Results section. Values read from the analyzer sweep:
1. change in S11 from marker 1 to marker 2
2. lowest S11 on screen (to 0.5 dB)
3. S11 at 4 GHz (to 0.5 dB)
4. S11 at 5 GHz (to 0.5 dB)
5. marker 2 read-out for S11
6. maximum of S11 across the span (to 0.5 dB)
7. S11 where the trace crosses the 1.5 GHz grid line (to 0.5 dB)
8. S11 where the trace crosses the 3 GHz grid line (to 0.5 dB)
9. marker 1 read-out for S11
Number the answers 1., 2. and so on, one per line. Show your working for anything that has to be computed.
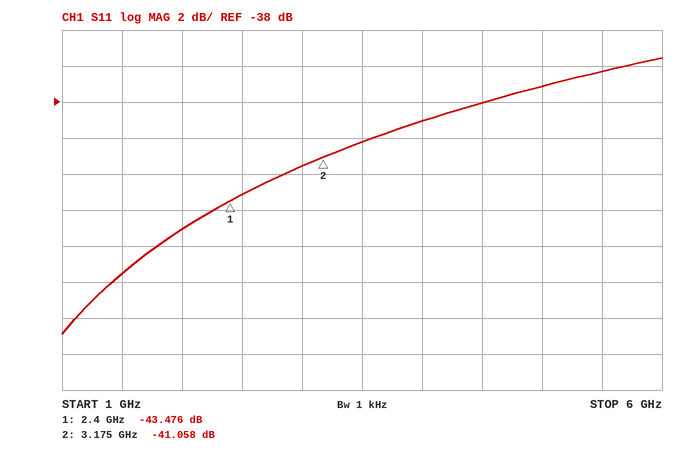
1. -41.058 − (-43.476) = 2.418 dB
2. -51.0 dB
3. -39.0 dB
4. -37.0 dB
5. -41.058 dB
6. -35.5 dB
7. -47.5 dB
8. -41.5 dB
9. -43.476 dB
